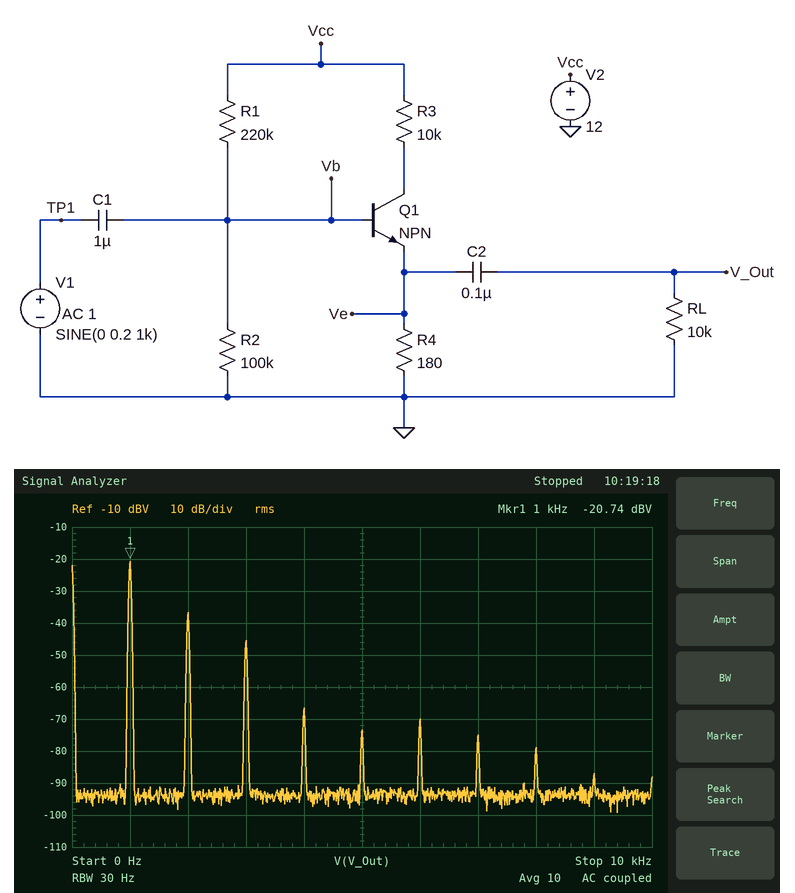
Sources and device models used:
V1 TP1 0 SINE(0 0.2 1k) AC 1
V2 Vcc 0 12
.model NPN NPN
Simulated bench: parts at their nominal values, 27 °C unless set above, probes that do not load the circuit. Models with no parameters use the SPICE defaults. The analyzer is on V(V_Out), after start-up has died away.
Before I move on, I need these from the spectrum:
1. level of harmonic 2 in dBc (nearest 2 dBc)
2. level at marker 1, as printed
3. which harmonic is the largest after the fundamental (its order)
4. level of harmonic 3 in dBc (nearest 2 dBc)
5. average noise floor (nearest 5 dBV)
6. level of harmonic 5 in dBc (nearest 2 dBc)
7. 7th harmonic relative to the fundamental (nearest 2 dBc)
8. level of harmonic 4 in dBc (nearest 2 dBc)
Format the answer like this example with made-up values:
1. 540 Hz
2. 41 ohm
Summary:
1. -16 dBc
2. -20.74 dBV
3. 2
4. -24 dBc
5. -95 dBV
6. -52 dBc
7. -54 dBc
8. -46 dBc
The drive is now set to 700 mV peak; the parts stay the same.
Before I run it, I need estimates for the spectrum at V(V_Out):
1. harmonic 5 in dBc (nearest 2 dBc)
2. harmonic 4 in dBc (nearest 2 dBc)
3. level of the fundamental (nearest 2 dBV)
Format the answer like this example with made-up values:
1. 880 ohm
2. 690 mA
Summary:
1. -24 dBc
2. -22 dBc
3. -22 dBV
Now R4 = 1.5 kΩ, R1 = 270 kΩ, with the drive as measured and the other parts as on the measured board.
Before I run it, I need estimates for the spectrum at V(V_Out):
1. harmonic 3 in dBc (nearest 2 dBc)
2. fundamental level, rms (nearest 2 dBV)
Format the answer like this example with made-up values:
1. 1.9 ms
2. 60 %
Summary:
1. -54 dBc
2. -18 dBV
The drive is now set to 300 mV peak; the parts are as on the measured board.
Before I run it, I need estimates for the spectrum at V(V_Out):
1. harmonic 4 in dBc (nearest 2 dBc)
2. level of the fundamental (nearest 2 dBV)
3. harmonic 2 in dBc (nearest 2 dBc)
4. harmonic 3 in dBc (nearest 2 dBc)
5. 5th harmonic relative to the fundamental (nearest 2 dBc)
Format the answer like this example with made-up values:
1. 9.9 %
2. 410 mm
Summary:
1. -24 dBc
2. -20 dBV
3. -8 dBc
4. -32 dBc
5. -48 dBc
